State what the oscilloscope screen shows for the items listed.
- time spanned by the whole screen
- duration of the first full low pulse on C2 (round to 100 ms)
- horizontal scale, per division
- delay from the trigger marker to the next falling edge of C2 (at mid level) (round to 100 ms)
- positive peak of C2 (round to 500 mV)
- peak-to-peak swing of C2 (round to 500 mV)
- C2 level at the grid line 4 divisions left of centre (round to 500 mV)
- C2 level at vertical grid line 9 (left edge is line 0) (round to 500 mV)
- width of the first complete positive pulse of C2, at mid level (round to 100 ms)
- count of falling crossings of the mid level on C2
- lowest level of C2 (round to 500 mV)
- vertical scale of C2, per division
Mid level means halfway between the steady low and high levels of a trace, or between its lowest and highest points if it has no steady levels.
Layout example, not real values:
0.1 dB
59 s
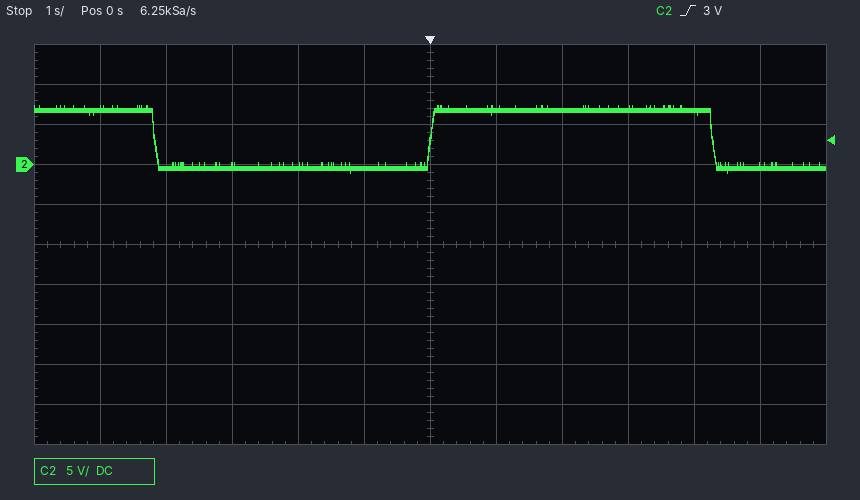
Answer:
12 s
4.2 s
1 s
4.3 s
7.5 V
8.5 V
-500 mV
7.0 V
4.3 s
2
-1.0 V
5 V
